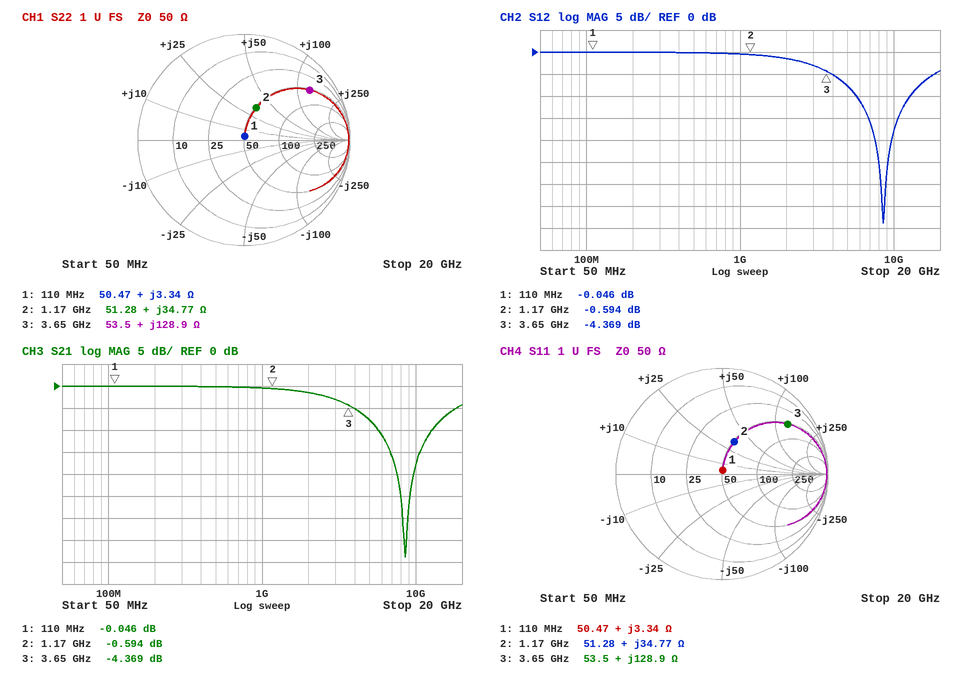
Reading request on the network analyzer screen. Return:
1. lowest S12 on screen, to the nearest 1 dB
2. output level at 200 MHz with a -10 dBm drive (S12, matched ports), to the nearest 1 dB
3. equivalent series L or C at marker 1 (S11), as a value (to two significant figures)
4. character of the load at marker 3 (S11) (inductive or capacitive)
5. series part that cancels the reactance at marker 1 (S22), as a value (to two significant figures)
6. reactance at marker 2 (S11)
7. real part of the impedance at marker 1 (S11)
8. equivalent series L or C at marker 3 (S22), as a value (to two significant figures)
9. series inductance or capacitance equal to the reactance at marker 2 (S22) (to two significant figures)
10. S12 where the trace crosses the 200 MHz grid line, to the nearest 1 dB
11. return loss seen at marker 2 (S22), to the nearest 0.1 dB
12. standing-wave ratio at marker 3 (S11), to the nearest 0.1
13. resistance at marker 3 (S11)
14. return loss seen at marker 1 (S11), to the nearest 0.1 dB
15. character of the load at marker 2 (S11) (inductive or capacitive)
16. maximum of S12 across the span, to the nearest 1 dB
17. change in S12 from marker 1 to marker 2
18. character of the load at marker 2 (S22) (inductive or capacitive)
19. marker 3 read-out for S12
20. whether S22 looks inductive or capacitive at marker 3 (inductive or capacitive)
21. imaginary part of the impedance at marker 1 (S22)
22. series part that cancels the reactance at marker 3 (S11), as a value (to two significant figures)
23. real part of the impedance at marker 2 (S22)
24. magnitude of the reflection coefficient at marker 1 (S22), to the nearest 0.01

-39 dB
-10 dBm
4.8 nH
inductive
430 pF
+34.77 Ω
50.47 Ω
5.6 nH
4.7 nH
0 dB
9.8 dB
8.1
53.5 Ω
29.5 dB
inductive
0 dB
-0.548 dB
inductive
-4.369 dB
inductive
+3.34 Ω
340 fF
51.28 Ω
0.03
